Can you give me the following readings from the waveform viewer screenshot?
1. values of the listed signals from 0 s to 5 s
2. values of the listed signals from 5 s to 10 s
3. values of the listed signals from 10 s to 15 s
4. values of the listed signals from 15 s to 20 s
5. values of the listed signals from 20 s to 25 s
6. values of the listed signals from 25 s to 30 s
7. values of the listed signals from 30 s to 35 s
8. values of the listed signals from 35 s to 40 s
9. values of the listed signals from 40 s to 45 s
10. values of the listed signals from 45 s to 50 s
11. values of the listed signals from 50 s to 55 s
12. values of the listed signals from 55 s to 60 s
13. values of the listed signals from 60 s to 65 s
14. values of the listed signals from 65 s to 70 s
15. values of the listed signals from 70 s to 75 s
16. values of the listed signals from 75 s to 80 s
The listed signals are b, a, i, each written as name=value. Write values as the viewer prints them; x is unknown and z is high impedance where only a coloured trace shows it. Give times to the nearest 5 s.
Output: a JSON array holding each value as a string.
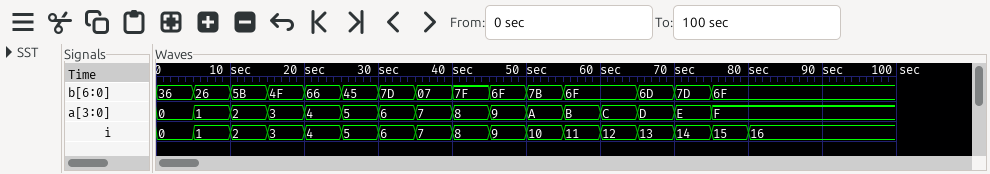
["b=36, a=0, i=0", "b=26, a=1, i=1", "b=5B, a=2, i=2", "b=4F, a=3, i=3", "b=66, a=4, i=4", "b=45, a=5, i=5", "b=7D, a=6, i=6", "b=07, a=7, i=7", "b=7F, a=8, i=8", "b=6F, a=9, i=9", "b=7B, a=A, i=10", "b=6F, a=B, i=11", "b=6F, a=C, i=12", "b=6D, a=D, i=13", "b=7D, a=E, i=14", "b=6F, a=F, i=15"]
